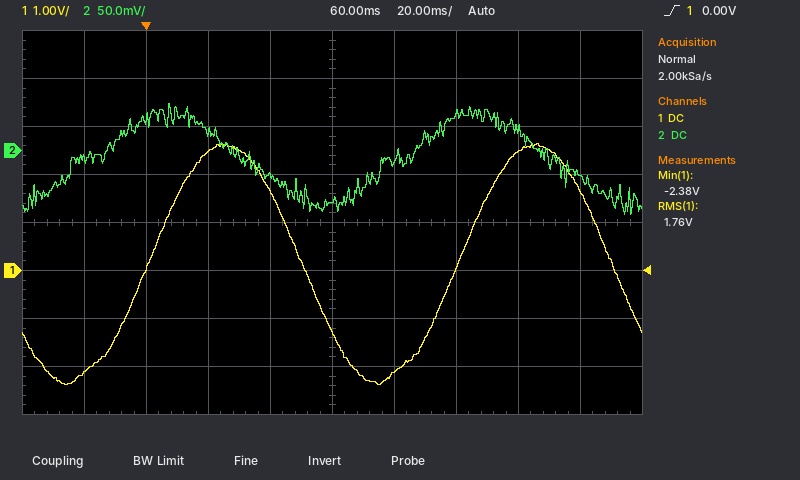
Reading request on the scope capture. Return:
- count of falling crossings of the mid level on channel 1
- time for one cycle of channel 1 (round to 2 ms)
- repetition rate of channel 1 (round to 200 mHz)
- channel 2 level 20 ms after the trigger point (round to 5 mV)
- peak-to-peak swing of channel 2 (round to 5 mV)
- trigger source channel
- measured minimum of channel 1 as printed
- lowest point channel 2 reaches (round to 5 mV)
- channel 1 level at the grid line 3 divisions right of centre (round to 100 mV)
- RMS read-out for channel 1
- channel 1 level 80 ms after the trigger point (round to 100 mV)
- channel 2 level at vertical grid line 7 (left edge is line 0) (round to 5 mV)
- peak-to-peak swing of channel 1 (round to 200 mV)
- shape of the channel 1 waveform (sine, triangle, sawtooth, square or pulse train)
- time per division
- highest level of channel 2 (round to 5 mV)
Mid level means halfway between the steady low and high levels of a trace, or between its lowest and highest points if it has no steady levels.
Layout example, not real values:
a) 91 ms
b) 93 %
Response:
a) 2
b) 100 ms
c) 10.0 Hz
d) 20 mV
e) 115 mV
f) channel 1
g) -2.38 V
h) -65 mV
i) 2.5 V
j) 1.76 V
k) -2.1 V
l) 40 mV
m) 5.0 V
n) sine
o) 20 ms
p) 50 mV
